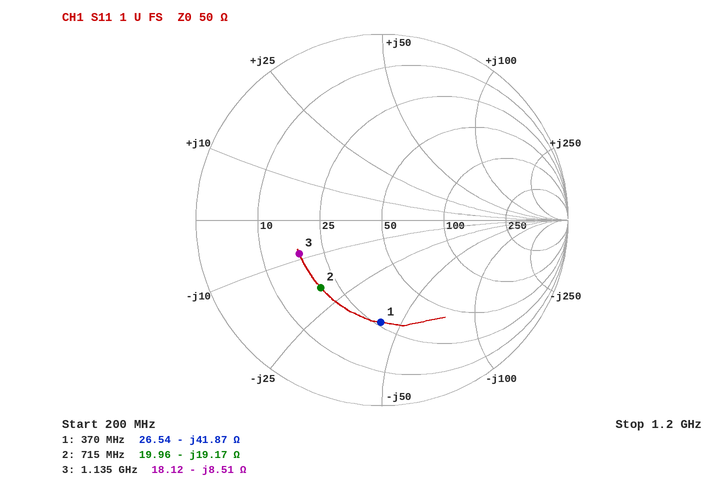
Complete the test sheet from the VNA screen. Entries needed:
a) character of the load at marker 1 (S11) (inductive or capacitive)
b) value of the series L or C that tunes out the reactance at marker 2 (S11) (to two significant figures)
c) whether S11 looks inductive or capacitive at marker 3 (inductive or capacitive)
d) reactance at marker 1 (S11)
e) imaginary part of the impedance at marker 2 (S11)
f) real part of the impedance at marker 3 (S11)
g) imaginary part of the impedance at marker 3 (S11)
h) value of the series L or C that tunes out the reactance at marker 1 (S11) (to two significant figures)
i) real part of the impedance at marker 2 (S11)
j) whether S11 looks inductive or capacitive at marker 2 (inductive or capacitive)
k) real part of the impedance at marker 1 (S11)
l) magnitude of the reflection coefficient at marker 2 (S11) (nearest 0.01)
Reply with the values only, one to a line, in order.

capacitive
4.3 nH
capacitive
-41.87 Ω
-19.17 Ω
18.12 Ω
-8.51 Ω
18 nH
19.96 Ω
capacitive
26.54 Ω
0.49
